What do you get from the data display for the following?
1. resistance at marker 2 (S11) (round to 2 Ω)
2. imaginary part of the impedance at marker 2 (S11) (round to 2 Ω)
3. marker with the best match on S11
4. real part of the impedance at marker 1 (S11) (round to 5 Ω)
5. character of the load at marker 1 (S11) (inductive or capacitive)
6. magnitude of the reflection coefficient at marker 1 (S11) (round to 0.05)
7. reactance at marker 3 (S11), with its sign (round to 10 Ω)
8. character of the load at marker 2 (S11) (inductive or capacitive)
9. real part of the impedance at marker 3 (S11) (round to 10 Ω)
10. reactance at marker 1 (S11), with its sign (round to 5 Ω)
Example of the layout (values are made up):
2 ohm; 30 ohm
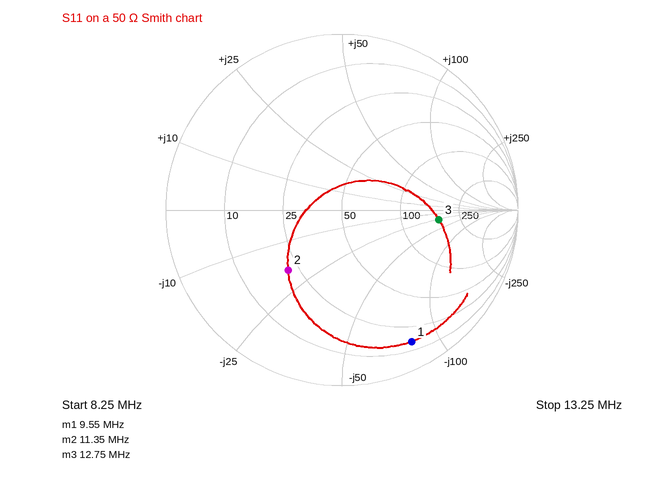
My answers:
22 Ω; -18 Ω; marker 2; 15 Ω; capacitive; 0.85; -30 Ω; capacitive; 170 Ω; -80 Ω
